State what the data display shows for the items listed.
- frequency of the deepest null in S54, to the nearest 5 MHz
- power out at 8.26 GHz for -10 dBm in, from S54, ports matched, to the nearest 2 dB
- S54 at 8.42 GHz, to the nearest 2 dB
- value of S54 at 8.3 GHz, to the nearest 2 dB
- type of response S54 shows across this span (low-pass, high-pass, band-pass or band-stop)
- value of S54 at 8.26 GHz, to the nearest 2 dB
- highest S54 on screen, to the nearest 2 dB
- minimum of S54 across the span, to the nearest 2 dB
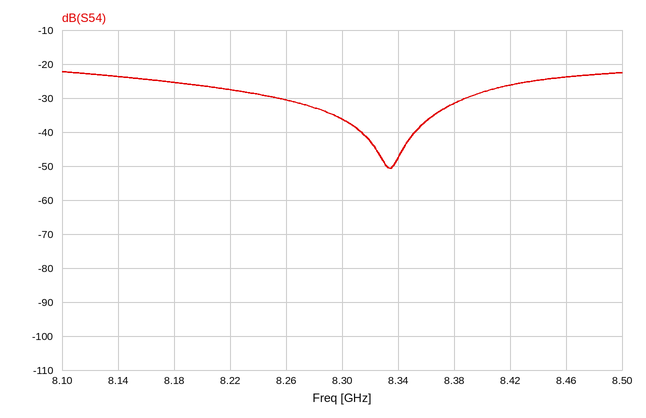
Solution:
8.335 GHz
-40 dBm
-26 dB
-36 dB
band-stop
-30 dB
-22 dB
-50 dB
